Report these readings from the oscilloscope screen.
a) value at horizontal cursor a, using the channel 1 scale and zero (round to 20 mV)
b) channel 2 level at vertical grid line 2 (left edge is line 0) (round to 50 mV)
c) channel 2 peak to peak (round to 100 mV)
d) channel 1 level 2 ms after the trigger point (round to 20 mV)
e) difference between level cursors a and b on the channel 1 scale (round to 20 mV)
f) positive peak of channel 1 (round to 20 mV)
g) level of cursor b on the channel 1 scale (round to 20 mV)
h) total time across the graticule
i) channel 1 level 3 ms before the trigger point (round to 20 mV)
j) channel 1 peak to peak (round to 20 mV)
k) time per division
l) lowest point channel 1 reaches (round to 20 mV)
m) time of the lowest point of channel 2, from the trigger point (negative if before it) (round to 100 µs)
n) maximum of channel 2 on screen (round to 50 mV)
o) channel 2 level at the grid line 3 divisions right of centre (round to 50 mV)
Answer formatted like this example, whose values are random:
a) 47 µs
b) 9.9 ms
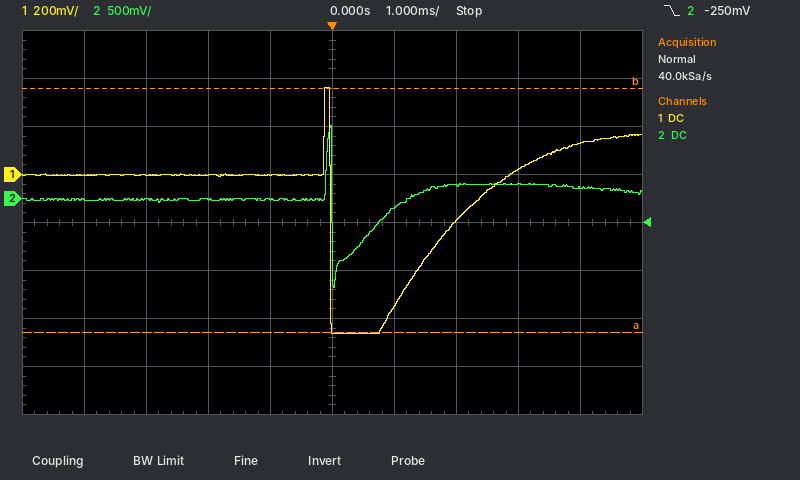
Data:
a) -660 mV
b) 0 mV
c) 1.70 V
d) -200 mV
e) 1.02 V
f) 360 mV
g) 360 mV
h) 10 ms
i) 0 mV
j) 1.02 V
k) 1 ms
l) -660 mV
m) 0.0 ms
n) 750 mV
o) 150 mV
